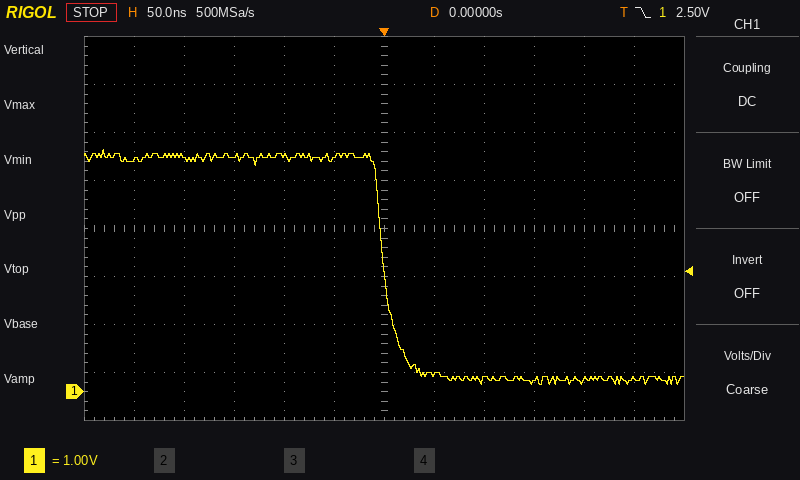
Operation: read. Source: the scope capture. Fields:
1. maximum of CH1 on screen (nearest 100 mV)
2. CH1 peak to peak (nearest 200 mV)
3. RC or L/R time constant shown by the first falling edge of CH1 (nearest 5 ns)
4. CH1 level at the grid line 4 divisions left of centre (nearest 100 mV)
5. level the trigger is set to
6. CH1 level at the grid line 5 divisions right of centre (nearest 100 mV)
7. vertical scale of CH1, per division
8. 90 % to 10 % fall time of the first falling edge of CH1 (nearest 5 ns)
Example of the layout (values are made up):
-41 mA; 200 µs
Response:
5.0 V; 4.8 V; 15 ns; 4.9 V; 2.50 V; 300 mV; 1 V; 30 ns
